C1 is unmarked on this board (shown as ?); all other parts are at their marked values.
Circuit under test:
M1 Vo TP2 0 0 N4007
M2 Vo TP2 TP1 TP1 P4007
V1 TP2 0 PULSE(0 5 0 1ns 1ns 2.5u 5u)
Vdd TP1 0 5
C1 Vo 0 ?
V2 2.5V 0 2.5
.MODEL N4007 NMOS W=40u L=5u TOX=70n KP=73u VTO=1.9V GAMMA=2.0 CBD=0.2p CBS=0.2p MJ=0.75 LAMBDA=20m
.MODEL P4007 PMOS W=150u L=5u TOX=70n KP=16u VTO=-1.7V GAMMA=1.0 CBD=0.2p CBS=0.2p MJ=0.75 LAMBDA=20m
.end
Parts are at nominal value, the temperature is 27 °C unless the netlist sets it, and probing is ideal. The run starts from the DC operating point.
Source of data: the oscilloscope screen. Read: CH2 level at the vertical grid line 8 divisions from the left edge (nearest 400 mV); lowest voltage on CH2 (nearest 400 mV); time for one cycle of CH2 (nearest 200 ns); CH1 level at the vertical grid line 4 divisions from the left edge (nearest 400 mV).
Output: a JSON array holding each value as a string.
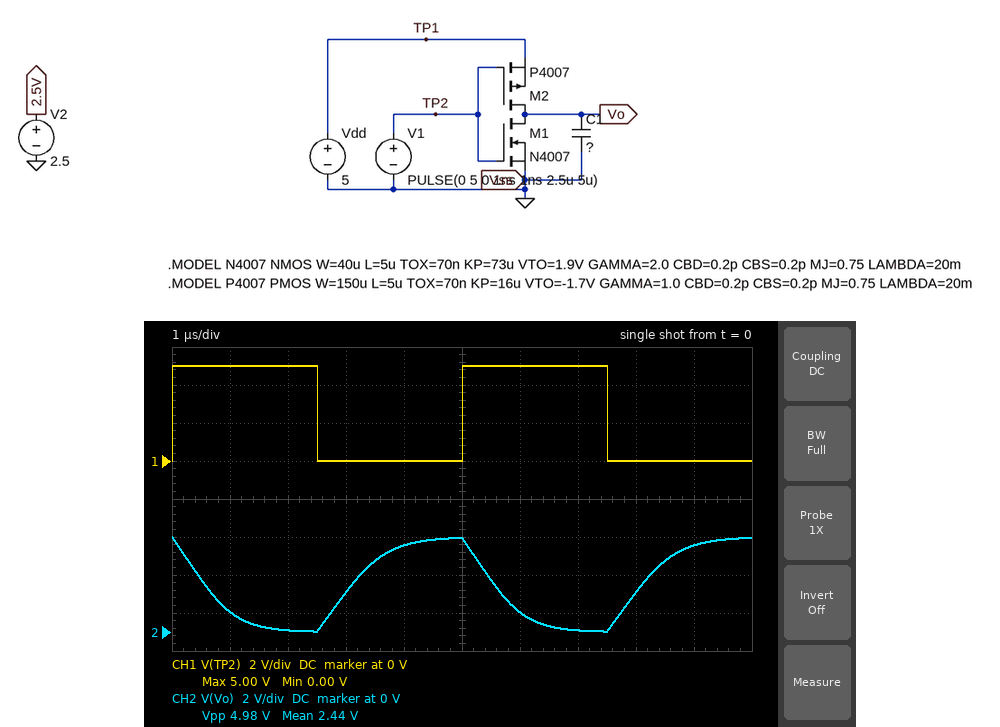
["2.0 V", "0 V", "5.0 µs", "0 V"]
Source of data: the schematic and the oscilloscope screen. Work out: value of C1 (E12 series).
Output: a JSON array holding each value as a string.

["680 pF"]
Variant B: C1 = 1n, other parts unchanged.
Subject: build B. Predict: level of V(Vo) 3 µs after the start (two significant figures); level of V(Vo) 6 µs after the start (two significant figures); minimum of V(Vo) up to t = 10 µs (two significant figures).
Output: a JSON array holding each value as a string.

["1.6 V", "1.8 V", "160 mV"]
